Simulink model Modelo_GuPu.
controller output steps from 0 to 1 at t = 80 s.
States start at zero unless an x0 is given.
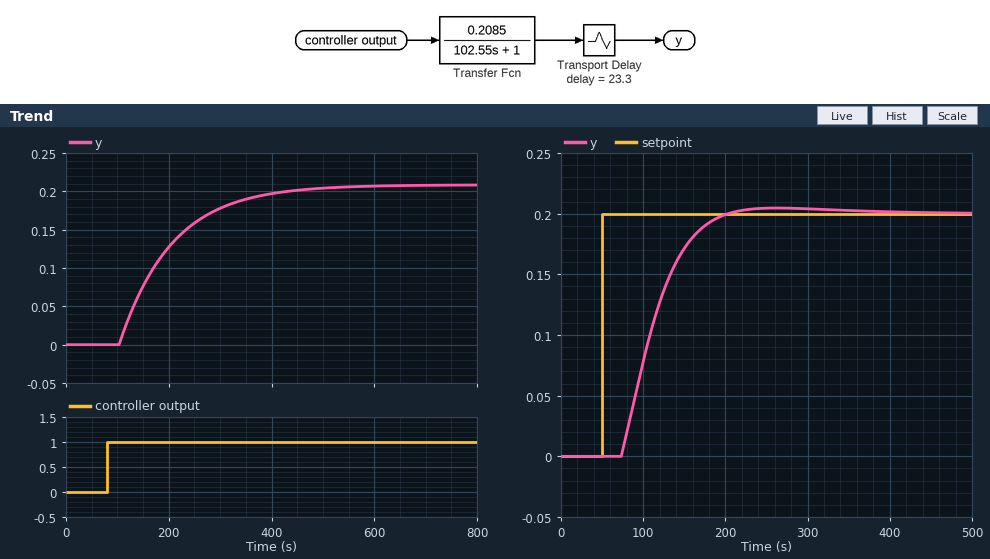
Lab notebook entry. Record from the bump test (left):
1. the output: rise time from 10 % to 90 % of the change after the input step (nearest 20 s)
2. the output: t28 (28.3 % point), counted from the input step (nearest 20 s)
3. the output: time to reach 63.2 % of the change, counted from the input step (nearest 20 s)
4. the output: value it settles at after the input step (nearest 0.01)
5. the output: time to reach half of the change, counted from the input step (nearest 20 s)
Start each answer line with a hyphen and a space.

- 220 s
- 60 s
- 120 s
- 0.21
- 100 s
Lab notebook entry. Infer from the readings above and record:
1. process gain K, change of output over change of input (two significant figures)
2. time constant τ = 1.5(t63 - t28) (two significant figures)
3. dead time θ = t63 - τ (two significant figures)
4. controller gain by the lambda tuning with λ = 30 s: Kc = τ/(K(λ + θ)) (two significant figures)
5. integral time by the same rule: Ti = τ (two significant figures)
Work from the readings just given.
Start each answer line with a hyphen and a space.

- 0.21
- 90 s
- 30 s
- 7.1
- 90 s
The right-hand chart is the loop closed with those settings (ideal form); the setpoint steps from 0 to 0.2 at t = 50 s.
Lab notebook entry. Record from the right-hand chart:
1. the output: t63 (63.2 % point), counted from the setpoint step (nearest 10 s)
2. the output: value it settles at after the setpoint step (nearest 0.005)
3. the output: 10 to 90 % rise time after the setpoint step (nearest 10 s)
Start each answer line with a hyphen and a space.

- 70 s
- 0.200
- 80 s
